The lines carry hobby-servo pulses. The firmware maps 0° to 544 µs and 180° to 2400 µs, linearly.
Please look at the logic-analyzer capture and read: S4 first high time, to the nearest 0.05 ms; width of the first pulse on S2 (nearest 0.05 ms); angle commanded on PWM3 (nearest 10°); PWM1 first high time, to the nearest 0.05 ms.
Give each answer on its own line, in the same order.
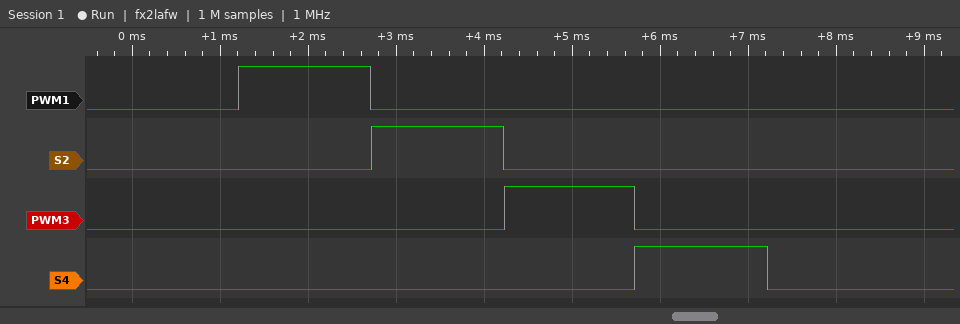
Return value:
1.50 ms
1.50 ms
90°
1.50 ms
